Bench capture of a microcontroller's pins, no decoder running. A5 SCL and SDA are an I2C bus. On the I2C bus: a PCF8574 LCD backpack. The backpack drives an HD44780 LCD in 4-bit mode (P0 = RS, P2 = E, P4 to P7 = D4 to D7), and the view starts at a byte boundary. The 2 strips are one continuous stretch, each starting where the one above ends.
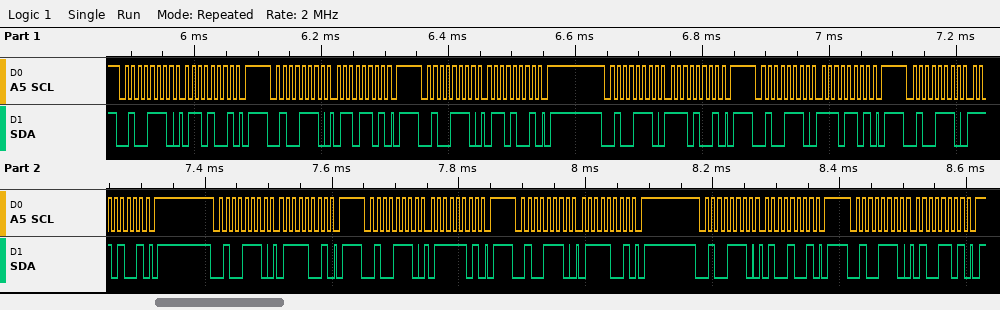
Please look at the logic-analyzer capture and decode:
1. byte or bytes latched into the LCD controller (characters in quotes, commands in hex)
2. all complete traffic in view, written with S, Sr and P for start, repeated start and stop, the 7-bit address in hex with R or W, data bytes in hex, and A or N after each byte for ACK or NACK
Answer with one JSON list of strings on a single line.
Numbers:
["'n'", "S 27W A 69 A P S 27W A 6D A P S 27W A 69 A P S 27W A E9 A P S 27W A ED A P S 27W A E9 A P S 27W A 79 A P S 27W A 7D A P S 27W A 79 A P S 27W A 49 A P S 27W A 4D A P"]
